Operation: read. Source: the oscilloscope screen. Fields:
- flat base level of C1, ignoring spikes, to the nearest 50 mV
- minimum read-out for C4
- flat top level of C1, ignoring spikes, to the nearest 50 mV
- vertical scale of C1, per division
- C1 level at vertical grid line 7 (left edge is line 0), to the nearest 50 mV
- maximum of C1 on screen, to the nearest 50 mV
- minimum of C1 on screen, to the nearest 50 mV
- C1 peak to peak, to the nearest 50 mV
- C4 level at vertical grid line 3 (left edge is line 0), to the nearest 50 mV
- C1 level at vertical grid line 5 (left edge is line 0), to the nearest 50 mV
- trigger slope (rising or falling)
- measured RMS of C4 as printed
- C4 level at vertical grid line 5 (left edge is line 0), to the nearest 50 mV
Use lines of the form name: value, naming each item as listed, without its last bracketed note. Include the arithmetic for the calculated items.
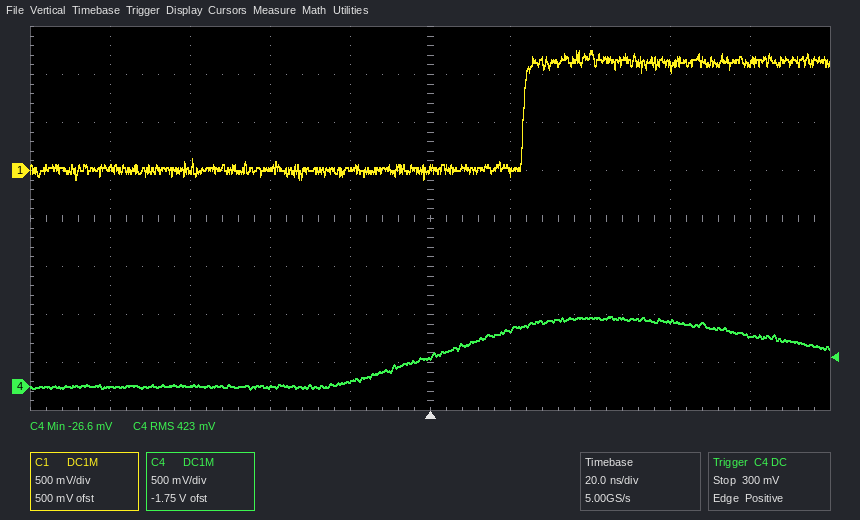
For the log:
flat base level of C1, ignoring spikes, to the nearest 50 mV: 0 mV
minimum read-out for C4: -26.6 mV
flat top level of C1, ignoring spikes, to the nearest 50 mV: 1.15 V
vertical scale of C1, per division: 500 mV
C1 level at vertical grid line 7 (left edge is line 0), to the nearest 50 mV: 1.20 V
maximum of C1 on screen, to the nearest 50 mV: 1.25 V
minimum of C1 on screen, to the nearest 50 mV: -100 mV
C1 peak to peak, to the nearest 50 mV: 1.25 V − (-100 mV) = 1.35 V
C4 level at vertical grid line 3 (left edge is line 0), to the nearest 50 mV: 0 mV
C1 level at vertical grid line 5 (left edge is line 0), to the nearest 50 mV: 0 mV
trigger slope: rising
measured RMS of C4 as printed: 423 mV
C4 level at vertical grid line 5 (left edge is line 0), to the nearest 50 mV: 300 mV
